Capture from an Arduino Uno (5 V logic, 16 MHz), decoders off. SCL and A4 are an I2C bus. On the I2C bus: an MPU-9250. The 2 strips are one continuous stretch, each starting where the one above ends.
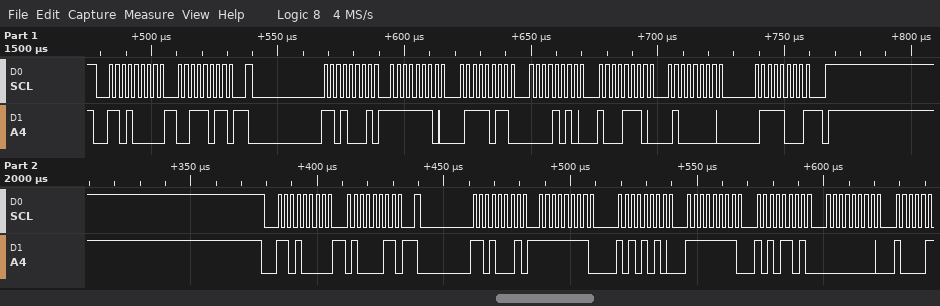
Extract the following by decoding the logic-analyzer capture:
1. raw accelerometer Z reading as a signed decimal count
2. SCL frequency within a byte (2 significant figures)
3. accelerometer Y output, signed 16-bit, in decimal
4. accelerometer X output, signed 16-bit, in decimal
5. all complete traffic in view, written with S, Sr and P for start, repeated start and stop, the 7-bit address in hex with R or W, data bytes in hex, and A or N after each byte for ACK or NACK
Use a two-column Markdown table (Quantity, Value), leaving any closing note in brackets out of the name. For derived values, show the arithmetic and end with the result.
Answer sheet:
| Quantity | Value |
|---|---|
| raw accelerometer Z reading as a signed decimal count | 0x4078 = 16504 |
| SCL frequency within a byte | 400 kHz |
| accelerometer Y output, signed 16-bit, in decimal | 0x0A8E = 2702 |
| accelerometer X output, signed 16-bit, in decimal | 0xFE7B = -389 |
| all complete traffic in view, written with S, Sr and P for start, repeated start and stop, the 7-bit address in hex with R or W, data bytes in hex, and A or N after each byte for ACK or NACK | S 68W A 3B A Sr 68R A FE A 7B A 0A A 8E A 40 A 78 N P S 68W A 43 A Sr 68R A FF A AA A FF A AD A 00 A |
